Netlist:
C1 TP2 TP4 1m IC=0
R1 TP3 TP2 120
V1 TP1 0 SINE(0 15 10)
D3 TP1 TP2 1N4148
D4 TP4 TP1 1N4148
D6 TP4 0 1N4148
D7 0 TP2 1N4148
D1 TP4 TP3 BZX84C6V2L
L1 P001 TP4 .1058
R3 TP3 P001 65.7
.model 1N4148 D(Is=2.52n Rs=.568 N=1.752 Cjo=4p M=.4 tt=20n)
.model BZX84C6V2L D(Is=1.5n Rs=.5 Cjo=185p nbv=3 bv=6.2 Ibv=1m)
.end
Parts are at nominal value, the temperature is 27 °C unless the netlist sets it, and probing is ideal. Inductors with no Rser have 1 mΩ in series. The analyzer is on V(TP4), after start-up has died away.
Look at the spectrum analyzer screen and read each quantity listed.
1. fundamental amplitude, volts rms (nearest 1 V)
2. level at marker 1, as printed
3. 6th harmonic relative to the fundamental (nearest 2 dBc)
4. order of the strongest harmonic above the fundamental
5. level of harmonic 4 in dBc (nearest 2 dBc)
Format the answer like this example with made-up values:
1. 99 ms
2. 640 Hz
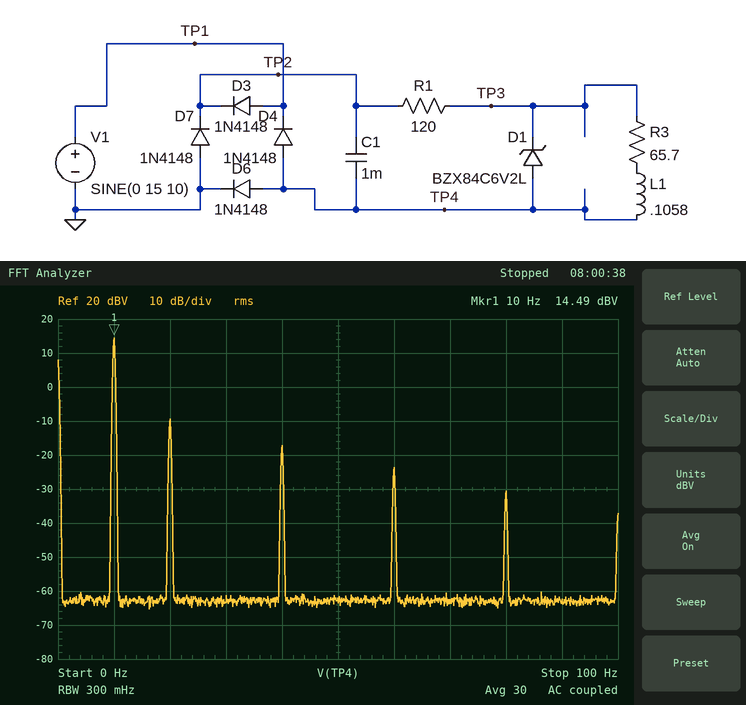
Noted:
1. 5 V
2. 14.49 dBV
3. -38 dBc
4. 2
5. -32 dBc
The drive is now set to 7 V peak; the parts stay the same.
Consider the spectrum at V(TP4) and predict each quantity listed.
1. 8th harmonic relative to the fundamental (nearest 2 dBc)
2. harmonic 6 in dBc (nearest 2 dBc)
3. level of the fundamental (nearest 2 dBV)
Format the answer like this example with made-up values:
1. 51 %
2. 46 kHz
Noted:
1. -46 dBc
2. -40 dBc
3. 8 dBV
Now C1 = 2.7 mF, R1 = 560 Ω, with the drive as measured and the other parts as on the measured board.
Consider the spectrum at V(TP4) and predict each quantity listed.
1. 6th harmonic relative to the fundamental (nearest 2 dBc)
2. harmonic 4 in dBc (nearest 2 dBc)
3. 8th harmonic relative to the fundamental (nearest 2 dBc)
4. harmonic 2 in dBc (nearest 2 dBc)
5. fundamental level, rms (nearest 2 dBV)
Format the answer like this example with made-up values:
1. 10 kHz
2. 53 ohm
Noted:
1. -54 dBc
2. -48 dBc
3. -58 dBc
4. -42 dBc
5. 14 dBV
